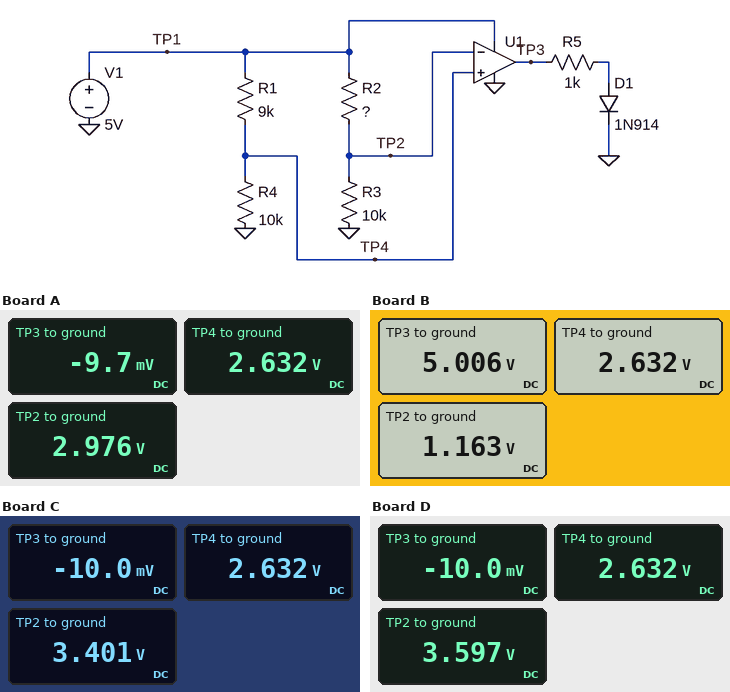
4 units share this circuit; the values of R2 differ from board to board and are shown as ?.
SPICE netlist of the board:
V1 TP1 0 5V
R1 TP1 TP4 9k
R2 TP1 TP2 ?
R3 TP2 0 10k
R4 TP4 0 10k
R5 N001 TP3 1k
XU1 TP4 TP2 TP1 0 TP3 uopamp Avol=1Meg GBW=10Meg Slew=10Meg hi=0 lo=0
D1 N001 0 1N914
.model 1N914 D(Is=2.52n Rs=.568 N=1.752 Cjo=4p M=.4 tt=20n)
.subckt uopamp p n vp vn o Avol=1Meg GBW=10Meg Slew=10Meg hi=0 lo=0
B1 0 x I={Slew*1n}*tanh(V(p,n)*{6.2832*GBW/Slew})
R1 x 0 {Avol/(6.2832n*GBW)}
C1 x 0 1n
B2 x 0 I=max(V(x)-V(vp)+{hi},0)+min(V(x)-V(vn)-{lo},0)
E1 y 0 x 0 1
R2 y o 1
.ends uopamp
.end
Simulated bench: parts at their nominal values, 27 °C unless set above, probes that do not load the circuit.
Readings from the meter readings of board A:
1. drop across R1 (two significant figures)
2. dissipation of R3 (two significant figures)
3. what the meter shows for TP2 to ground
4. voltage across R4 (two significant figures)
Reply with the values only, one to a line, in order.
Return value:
2.4 V
890 µW
2.976 V
2.6 V
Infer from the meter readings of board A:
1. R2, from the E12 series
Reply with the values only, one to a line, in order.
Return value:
6.8 kΩ
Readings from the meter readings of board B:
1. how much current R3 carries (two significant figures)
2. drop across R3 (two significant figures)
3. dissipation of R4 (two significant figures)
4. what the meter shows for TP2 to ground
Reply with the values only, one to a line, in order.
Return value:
120 µA
1.2 V
690 µW
1.163 V
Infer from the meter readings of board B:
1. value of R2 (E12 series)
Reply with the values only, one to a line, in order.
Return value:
33 kΩ
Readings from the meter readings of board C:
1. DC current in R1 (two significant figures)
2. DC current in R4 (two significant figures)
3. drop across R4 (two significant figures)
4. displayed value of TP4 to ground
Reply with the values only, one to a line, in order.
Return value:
260 µA
260 µA
2.6 V
2.632 V
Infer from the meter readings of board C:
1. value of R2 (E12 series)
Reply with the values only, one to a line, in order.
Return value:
4.7 kΩ
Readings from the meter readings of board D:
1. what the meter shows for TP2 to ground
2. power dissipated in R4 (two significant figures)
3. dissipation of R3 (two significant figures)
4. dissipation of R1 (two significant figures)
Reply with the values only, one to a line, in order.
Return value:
3.597 V
690 µW
1.3 mW
620 µW
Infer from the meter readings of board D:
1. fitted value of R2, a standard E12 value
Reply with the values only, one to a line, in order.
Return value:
3.9 kΩ
